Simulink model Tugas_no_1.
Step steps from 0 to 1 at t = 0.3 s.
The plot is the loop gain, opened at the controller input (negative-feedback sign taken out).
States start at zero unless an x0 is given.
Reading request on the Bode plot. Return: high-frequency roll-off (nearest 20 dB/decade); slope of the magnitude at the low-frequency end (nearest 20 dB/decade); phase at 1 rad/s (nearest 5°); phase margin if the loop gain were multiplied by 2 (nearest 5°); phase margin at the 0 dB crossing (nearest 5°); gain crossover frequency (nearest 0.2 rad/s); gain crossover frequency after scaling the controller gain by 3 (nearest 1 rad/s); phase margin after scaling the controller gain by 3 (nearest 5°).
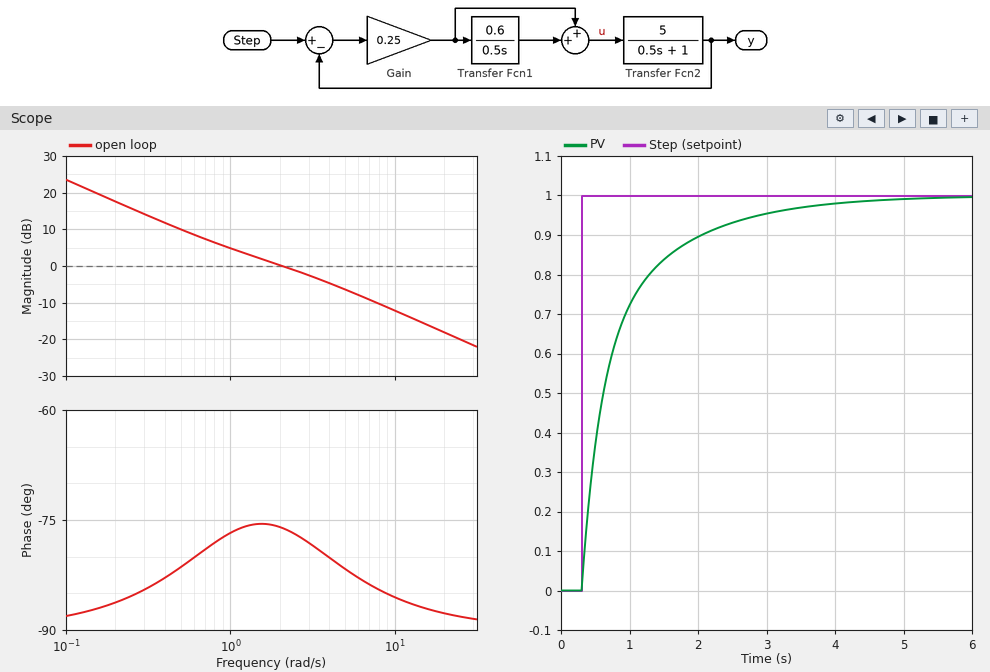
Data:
-20 dB/decade
-20 dB/decade
-75°
100°
105°
2.0 rad/s
7 rad/s
95°
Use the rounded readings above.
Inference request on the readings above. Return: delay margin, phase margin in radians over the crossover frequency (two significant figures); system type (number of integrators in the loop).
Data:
0.92 s
1
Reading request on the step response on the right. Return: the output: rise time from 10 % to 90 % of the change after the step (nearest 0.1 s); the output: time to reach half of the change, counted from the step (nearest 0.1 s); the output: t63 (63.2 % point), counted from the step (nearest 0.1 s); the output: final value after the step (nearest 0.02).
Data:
1.7 s
0.3 s
0.5 s
1.00
